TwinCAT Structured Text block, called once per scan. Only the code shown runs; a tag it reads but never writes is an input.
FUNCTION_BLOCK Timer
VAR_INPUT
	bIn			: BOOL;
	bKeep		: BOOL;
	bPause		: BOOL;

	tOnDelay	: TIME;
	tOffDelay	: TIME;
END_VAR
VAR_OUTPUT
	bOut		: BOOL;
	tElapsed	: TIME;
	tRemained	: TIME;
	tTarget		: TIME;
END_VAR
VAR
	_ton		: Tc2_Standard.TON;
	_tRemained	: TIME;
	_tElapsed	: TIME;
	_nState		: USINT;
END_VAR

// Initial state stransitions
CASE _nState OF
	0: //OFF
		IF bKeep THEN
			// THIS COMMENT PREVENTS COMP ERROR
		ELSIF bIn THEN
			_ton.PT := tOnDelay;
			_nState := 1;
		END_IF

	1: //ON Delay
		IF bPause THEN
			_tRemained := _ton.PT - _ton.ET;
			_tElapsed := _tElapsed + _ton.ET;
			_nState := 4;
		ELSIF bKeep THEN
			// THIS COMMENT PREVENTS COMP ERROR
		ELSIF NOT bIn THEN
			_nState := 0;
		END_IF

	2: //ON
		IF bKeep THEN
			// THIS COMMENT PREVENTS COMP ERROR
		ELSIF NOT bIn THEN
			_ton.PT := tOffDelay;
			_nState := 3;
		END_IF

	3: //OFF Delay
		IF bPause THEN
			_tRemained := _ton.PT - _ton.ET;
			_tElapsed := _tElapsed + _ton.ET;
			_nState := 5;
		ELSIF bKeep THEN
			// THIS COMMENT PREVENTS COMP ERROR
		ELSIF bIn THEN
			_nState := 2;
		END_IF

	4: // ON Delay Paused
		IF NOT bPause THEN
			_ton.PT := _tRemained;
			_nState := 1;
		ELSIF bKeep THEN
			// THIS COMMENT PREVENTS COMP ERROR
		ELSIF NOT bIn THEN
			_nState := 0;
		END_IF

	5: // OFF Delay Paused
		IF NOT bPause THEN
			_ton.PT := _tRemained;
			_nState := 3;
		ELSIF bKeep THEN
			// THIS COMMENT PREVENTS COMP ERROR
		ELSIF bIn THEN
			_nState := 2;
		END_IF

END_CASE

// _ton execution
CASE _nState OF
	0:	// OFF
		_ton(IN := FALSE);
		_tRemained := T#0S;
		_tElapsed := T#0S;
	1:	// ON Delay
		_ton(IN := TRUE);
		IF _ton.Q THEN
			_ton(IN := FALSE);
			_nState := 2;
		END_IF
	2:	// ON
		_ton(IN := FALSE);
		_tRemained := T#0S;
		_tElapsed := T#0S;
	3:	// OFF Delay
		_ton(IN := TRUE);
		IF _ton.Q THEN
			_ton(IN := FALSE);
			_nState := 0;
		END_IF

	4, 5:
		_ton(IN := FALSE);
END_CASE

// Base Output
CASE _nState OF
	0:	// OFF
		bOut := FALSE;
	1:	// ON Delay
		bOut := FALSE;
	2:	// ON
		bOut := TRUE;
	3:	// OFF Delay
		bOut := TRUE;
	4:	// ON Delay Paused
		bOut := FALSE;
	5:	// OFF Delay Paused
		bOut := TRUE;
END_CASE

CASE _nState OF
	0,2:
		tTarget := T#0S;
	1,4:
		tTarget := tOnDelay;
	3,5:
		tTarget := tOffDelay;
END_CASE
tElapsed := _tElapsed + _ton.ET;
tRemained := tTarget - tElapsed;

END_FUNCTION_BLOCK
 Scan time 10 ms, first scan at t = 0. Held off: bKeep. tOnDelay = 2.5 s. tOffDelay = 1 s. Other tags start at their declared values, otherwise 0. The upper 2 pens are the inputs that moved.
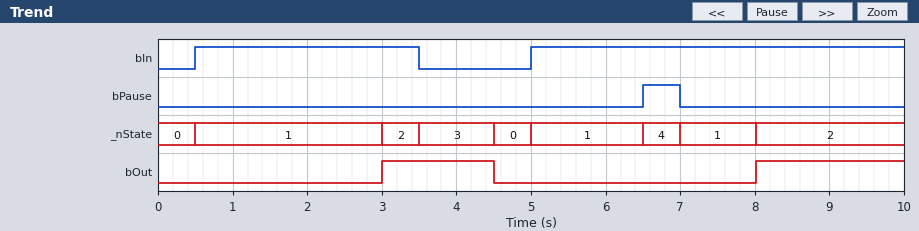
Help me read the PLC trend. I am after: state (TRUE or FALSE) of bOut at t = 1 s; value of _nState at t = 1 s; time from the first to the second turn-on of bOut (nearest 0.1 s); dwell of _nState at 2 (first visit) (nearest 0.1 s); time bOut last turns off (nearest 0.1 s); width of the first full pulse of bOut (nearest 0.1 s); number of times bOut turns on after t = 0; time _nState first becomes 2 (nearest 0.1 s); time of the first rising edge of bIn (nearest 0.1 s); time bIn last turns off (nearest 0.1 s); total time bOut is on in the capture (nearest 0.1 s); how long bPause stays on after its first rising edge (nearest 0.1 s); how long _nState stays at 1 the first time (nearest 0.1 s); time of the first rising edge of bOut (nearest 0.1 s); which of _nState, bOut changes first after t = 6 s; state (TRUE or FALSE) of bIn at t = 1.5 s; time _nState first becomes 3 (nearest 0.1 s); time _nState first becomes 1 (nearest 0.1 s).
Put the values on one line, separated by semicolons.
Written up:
FALSE; 1; 5.0 s; 0.5 s; 4.5 s; 1.5 s; 2; 3.0 s; 0.5 s; 3.5 s; 3.5 s; 0.5 s; 2.5 s; 3.0 s; _nState; TRUE; 3.5 s; 0.5 s
